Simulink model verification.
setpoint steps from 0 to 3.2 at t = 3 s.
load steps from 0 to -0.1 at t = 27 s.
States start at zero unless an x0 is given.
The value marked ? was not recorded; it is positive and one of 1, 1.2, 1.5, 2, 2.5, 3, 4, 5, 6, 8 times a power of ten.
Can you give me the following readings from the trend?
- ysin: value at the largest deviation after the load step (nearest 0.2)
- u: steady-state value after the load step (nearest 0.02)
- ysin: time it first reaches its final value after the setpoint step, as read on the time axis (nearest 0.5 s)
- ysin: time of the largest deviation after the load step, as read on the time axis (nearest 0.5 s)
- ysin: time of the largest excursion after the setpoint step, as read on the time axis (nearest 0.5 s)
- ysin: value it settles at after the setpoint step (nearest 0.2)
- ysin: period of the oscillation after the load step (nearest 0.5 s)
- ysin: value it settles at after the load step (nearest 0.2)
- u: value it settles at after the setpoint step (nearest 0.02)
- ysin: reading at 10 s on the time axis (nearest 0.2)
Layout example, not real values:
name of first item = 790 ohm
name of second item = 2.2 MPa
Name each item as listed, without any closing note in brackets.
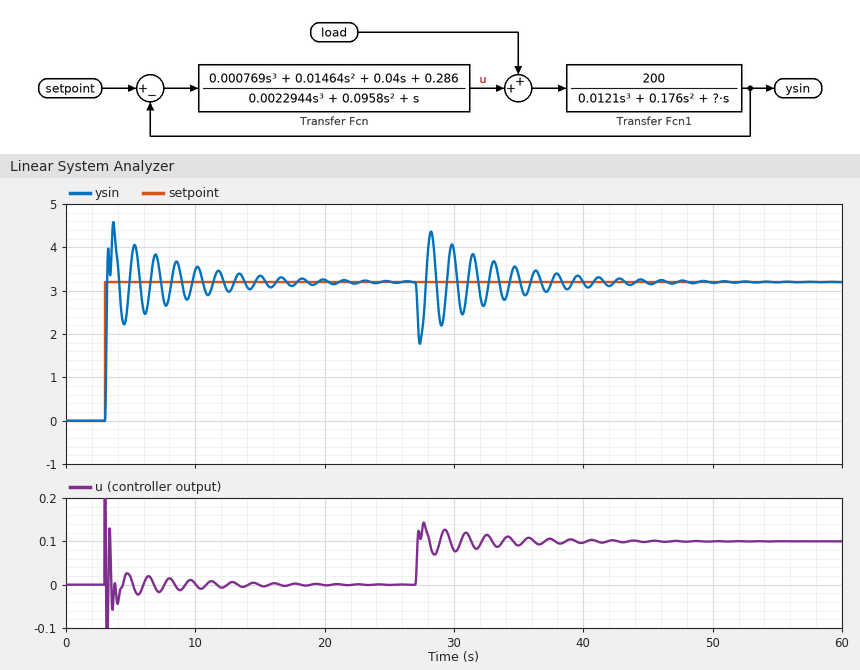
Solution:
ysin: value at the largest deviation after the load step = 1.8
u: steady-state value after the load step = 0.10
ysin: time it first reaches its final value after the setpoint step, as read on the time axis = 3.0 s
ysin: time of the largest deviation after the load step, as read on the time axis = 27.5 s
ysin: time of the largest excursion after the setpoint step, as read on the time axis = 3.5 s
ysin: value it settles at after the setpoint step = 3.2
ysin: period of the oscillation after the load step = 1.5 s
ysin: value it settles at after the load step = 3.2
u: value it settles at after the setpoint step = 0.00
ysin: reading at 10 s on the time axis = 3.4
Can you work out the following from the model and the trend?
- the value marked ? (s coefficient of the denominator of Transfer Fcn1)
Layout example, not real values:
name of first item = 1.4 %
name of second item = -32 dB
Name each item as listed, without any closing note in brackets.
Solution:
the value marked ? = 1.5
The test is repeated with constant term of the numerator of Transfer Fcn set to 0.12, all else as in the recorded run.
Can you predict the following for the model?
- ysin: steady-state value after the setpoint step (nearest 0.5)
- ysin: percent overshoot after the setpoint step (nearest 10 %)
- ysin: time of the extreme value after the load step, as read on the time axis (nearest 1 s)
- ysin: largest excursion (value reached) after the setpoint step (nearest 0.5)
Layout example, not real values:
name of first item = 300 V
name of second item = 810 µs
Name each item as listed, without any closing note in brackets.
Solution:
ysin: steady-state value after the setpoint step = 3.0
ysin: percent overshoot after the setpoint step = 20 %
ysin: time of the extreme value after the load step, as read on the time axis = 28 s
ysin: largest excursion (value reached) after the setpoint step = 4.0
